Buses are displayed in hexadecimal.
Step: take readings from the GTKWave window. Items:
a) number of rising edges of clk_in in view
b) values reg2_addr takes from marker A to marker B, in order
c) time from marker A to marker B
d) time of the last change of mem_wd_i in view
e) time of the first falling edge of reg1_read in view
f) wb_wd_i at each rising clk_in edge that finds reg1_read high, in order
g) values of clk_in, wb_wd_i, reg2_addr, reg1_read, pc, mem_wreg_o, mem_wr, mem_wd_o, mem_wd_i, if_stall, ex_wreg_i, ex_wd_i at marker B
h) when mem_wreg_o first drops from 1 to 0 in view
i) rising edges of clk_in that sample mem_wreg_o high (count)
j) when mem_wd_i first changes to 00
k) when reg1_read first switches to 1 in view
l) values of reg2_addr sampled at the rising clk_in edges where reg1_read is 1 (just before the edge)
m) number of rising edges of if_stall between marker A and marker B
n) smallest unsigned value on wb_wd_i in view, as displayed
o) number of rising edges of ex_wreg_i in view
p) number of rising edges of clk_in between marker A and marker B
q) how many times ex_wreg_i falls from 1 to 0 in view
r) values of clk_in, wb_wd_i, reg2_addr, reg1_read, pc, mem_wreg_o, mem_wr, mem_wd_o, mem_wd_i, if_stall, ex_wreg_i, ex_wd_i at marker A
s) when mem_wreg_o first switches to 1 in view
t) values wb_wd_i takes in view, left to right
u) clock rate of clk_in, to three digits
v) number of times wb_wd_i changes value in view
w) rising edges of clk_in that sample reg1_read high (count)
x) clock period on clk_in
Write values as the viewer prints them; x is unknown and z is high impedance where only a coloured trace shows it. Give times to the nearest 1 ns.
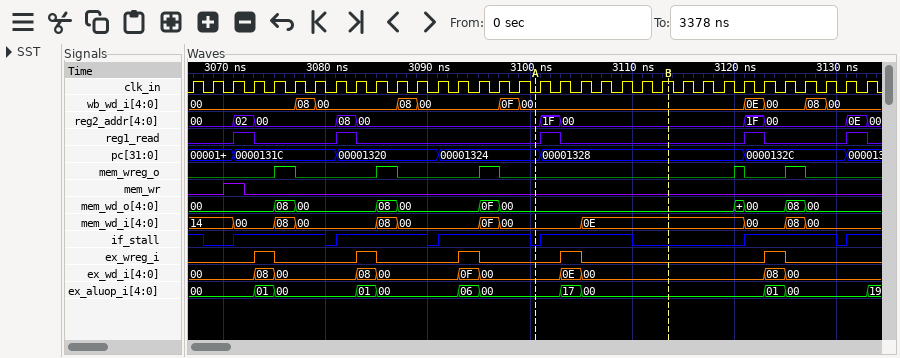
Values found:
34
00, 1F, 00
13 ns
3127 ns
3073 ns
00, 00, 00, 0E, 00
clk_in=1, wb_wd_i=00, reg2_addr=00, reg1_read=0, pc=00001328, mem_wreg_o=0, mem_wr=0, mem_wd_o=00, mem_wd_i=0E, if_stall=0, ex_wreg_i=0, ex_wd_i=00
3077 ns
5
3071 ns
3071 ns
02, 08, 1F, 1F, 0E
1
00
5
7
5
clk_in=0, wb_wd_i=00, reg2_addr=00, reg1_read=0, pc=00001324, mem_wreg_o=0, mem_wr=0, mem_wd_o=00, mem_wd_i=00, if_stall=0, ex_wreg_i=0, ex_wd_i=00
3075 ns
00, 08, 00, 08, 00, 0F, 00, 0E, 00, 08, 00
500 MHz
10
5
2 ns
